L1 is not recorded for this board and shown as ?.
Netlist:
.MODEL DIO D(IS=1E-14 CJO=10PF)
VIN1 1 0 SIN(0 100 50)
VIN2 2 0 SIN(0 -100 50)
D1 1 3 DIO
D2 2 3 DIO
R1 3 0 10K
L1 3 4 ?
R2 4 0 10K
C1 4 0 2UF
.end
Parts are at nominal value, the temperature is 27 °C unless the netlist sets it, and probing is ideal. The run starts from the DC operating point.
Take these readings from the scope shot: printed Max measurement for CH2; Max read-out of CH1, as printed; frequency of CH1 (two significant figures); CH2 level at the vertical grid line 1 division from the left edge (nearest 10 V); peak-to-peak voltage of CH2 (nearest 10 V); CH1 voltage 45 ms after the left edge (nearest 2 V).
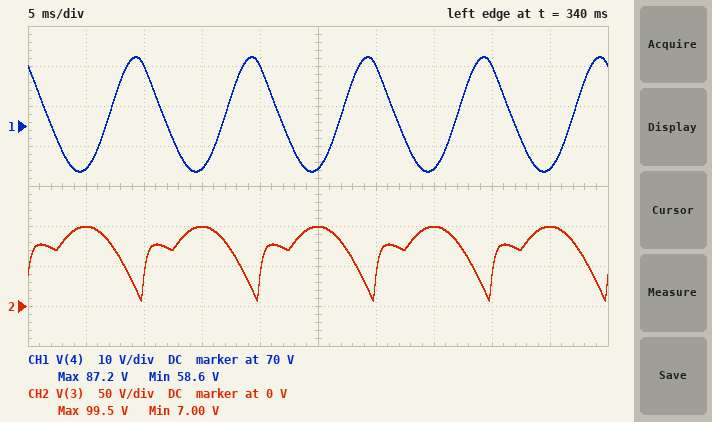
99.5 V
87.2 V
100 Hz
100 V
90 V
60 V
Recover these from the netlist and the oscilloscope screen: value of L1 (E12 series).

3.9 H
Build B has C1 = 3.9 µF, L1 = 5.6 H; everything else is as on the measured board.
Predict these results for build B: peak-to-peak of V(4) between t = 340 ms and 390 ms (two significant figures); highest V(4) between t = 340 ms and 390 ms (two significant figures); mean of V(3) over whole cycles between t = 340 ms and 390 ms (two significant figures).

11 V
70 V
64 V
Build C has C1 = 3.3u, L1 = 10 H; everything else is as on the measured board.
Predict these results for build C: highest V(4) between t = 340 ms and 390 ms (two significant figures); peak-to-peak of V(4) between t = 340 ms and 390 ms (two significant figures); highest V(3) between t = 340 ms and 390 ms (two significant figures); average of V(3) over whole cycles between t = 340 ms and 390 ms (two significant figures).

67 V
7.2 V
99 V
63 V
